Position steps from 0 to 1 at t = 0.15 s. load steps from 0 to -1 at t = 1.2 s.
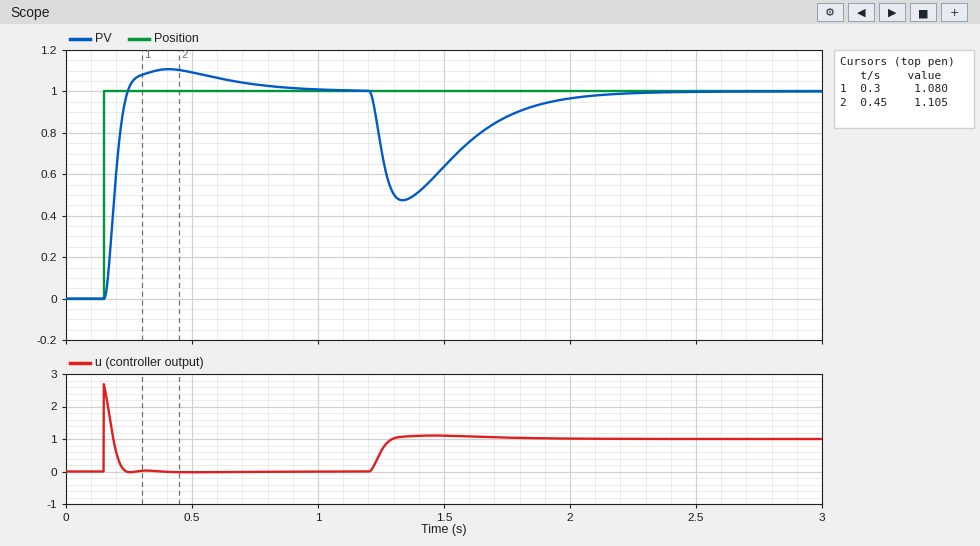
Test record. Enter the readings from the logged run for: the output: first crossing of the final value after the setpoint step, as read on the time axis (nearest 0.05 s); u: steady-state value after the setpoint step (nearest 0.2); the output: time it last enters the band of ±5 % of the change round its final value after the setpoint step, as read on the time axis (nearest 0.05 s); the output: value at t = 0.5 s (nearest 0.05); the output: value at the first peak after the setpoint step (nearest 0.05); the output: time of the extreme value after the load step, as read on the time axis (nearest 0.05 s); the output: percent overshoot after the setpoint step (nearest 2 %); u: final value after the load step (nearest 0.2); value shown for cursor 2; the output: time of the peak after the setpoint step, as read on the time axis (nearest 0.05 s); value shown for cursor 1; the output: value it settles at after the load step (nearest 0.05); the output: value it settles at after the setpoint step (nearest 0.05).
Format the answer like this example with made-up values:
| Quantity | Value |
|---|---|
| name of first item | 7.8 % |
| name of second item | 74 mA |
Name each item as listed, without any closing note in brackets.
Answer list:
| Quantity | Value |
|---|---|
| the output: first crossing of the final value after the setpoint step, as read on the time axis | 0.25 s |
| u: steady-state value after the setpoint step | 0.0 |
| the output: time it last enters the band of ±5 % of the change round its final value after the setpoint step, as read on the time axis | 0.65 s |
| the output: value at t = 0.5 s | 1.10 |
| the output: value at the first peak after the setpoint step | 1.10 |
| the output: time of the extreme value after the load step, as read on the time axis | 1.35 s |
| the output: percent overshoot after the setpoint step | 10 % |
| u: final value after the load step | 1.0 |
| value shown for cursor 2 | 1.105 |
| the output: time of the peak after the setpoint step, as read on the time axis | 0.40 s |
| value shown for cursor 1 | 1.080 |
| the output: value it settles at after the load step | 1.00 |
| the output: value it settles at after the setpoint step | 1.00 |
